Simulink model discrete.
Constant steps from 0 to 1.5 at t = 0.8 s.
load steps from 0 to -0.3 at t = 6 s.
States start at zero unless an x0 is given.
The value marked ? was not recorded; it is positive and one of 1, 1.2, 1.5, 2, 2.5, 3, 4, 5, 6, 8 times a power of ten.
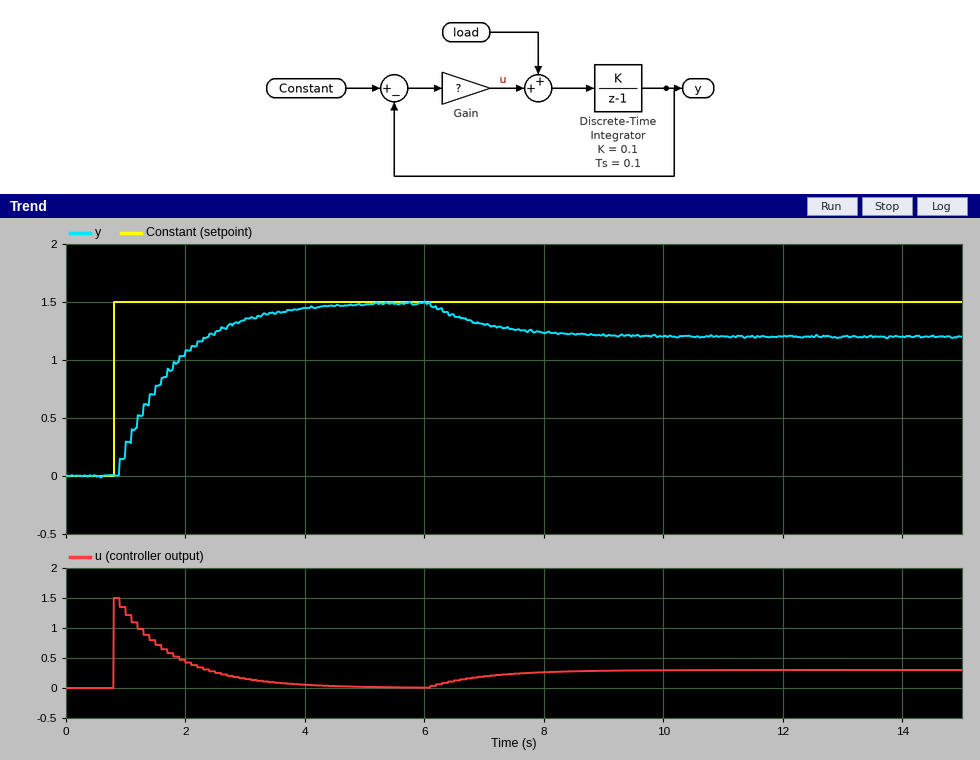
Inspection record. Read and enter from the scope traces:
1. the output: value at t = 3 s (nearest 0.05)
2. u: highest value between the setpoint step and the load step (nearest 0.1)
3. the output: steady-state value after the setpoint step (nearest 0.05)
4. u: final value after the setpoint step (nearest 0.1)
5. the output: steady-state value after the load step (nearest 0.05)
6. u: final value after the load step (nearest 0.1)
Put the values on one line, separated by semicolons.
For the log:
1.35; 1.5; 1.50; 0.0; 1.20; 0.3
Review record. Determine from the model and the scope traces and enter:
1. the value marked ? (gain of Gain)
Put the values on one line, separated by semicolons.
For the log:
1
